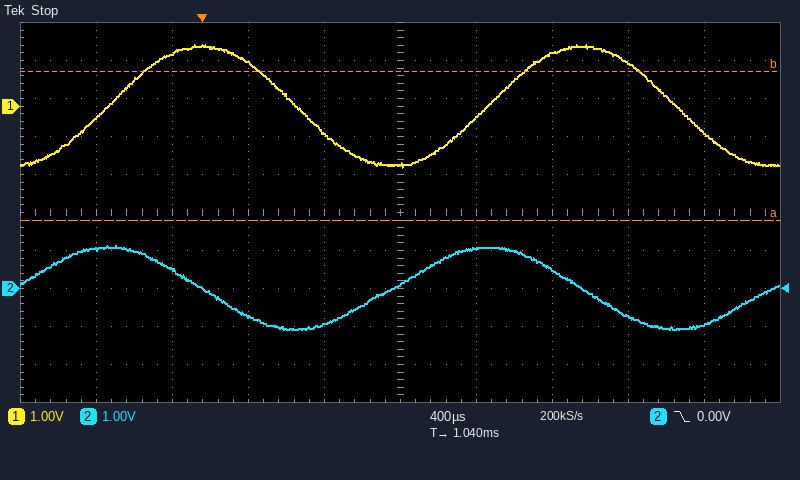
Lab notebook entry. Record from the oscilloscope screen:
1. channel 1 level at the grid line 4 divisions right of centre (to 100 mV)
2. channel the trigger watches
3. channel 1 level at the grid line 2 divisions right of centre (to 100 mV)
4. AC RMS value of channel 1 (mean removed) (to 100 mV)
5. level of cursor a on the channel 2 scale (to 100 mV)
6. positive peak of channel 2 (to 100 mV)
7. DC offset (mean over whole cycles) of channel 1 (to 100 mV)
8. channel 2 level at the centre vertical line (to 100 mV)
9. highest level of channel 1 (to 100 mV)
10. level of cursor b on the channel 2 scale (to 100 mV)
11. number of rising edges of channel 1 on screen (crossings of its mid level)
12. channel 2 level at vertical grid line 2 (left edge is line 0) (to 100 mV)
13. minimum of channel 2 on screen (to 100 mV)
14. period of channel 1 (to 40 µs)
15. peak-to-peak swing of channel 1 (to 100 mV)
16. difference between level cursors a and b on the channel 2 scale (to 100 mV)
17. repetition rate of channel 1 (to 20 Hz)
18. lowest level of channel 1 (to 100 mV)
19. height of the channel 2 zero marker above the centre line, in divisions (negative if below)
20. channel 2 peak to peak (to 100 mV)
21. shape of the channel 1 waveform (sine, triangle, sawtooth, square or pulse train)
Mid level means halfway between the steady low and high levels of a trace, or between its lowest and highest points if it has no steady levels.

-700 mV
channel 2
1.4 V
1.1 V
1.8 V
1.1 V
0.0 V
100 mV
1.6 V
5.7 V
2
500 mV
-1.1 V
2.00 ms
3.2 V
3.9 V
500 Hz
-1.6 V
-2.0 div
2.2 V
sine
